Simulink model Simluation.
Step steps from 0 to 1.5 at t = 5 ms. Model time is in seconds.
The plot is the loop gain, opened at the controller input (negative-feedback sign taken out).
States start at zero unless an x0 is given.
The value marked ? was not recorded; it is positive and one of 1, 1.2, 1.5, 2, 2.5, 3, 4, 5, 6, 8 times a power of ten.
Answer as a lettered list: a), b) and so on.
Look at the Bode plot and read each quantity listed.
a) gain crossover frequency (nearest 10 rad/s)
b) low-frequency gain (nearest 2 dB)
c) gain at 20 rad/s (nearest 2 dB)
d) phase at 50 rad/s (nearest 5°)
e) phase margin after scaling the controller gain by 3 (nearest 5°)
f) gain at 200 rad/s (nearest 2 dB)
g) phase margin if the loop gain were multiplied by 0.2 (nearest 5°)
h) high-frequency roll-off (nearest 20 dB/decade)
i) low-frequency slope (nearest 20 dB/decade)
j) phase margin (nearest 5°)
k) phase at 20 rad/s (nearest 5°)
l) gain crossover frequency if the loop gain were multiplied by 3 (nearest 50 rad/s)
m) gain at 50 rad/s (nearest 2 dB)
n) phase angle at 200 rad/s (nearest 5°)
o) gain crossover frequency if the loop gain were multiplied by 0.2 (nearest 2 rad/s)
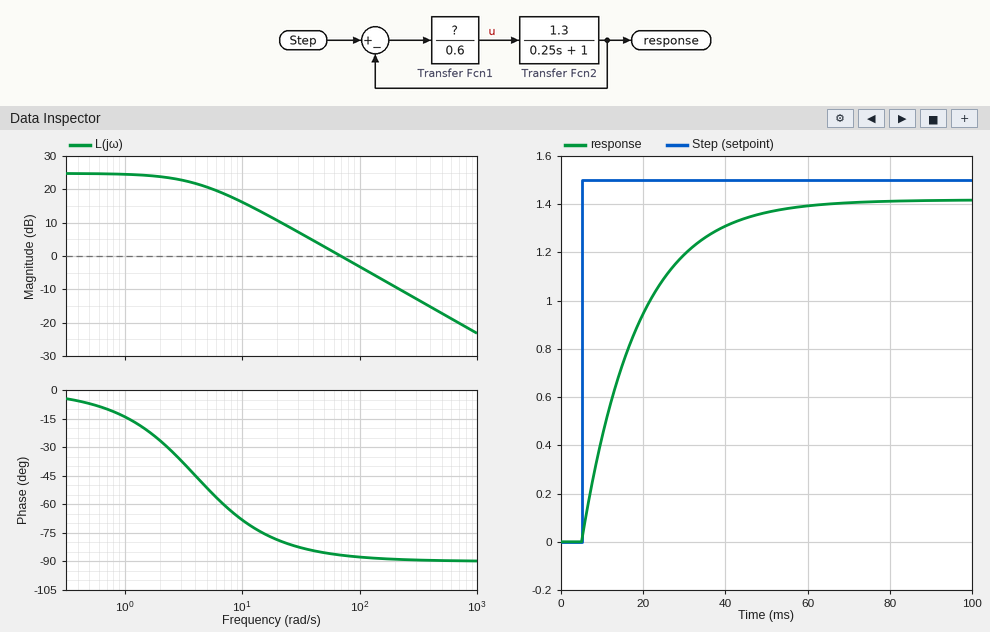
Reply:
a) 70 rad/s
b) 24 dB
c) 10 dB
d) -85°
e) 90°
f) -10 dB
g) 105°
h) -20 dB/decade
i) 0 dB/decade
j) 95°
k) -80°
l) 200 rad/s
m) 2 dB
n) -90°
o) 14 rad/s
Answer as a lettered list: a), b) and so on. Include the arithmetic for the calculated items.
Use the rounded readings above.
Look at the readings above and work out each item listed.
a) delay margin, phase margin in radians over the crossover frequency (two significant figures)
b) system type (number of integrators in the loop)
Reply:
a) 95 × π / 180 / 70 = 0.024 s
b) 0
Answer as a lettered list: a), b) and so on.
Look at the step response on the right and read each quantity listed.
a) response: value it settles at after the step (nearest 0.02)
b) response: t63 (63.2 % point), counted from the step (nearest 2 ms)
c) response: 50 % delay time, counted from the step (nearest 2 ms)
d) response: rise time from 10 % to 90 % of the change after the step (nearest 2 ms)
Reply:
a) 1.42
b) 14 ms
c) 10 ms
d) 30 ms
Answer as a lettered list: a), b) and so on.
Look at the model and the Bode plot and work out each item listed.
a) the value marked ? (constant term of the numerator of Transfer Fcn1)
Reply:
a) 8
